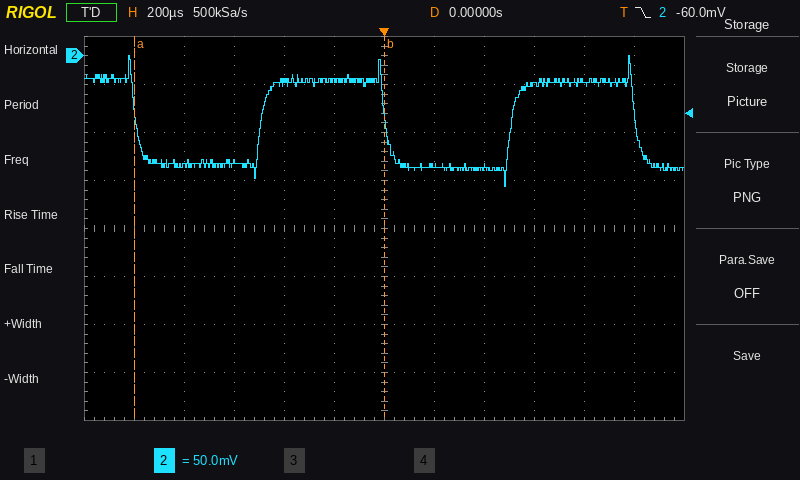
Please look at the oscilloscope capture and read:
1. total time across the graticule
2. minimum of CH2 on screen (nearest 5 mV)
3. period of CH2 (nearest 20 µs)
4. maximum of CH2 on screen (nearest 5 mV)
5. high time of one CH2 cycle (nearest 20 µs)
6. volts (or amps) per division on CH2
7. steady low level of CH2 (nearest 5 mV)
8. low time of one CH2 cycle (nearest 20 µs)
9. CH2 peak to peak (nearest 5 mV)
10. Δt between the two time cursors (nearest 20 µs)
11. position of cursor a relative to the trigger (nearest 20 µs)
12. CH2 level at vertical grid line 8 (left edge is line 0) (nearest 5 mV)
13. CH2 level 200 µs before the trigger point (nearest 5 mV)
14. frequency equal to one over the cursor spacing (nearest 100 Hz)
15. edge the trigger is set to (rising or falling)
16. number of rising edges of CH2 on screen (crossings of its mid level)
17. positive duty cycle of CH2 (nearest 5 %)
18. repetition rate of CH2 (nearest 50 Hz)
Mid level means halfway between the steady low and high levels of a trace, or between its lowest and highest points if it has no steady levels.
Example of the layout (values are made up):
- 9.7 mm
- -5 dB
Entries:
- 2.4 ms
- -135 mV
- 1.00 ms
- 0 mV
- 500 µs
- 50 mV
- -115 mV
- 500 µs
- 135 mV
- 1.00 ms
- -1.00 ms
- -115 mV
- -25 mV
- 1.0 kHz
- falling
- 2
- 50 %
- 1.00 kHz
